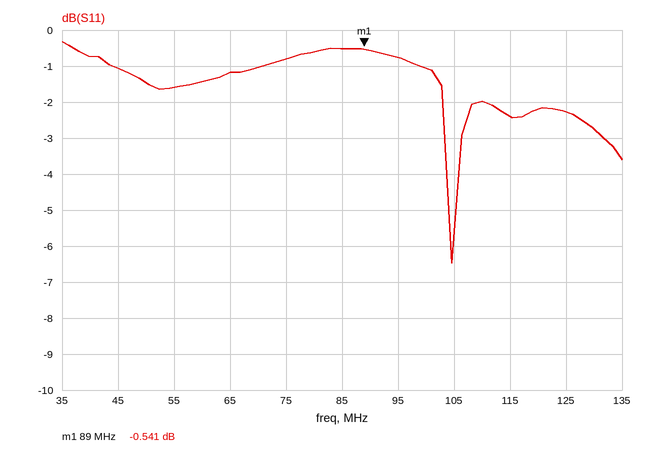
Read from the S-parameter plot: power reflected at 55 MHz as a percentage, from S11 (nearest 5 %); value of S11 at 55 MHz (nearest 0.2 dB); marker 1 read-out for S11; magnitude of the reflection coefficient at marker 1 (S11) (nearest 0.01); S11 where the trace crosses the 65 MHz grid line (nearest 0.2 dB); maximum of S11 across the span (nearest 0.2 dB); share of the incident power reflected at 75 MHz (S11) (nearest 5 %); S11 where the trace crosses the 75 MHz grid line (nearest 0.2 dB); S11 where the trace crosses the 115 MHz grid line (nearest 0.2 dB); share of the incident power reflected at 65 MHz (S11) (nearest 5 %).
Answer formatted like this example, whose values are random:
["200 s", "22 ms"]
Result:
["70 %", "-1.6 dB", "-0.541 dB", "0.94", "-1.2 dB", "-0.4 dB", "85 %", "-0.8 dB", "-2.4 dB", "75 %"]
